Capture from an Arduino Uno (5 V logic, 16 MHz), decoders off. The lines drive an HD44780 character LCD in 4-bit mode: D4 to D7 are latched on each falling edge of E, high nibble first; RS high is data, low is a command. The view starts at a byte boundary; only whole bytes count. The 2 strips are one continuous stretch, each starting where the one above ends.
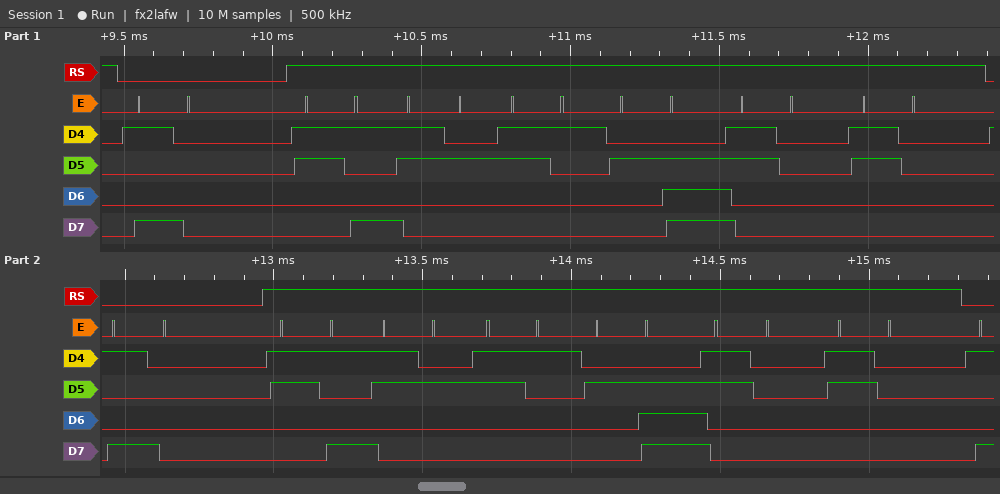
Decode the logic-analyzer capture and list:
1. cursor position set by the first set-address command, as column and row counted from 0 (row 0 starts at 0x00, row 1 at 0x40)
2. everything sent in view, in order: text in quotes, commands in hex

column 16, row 0
0x90 "921.00" 0x90 "921.00"
